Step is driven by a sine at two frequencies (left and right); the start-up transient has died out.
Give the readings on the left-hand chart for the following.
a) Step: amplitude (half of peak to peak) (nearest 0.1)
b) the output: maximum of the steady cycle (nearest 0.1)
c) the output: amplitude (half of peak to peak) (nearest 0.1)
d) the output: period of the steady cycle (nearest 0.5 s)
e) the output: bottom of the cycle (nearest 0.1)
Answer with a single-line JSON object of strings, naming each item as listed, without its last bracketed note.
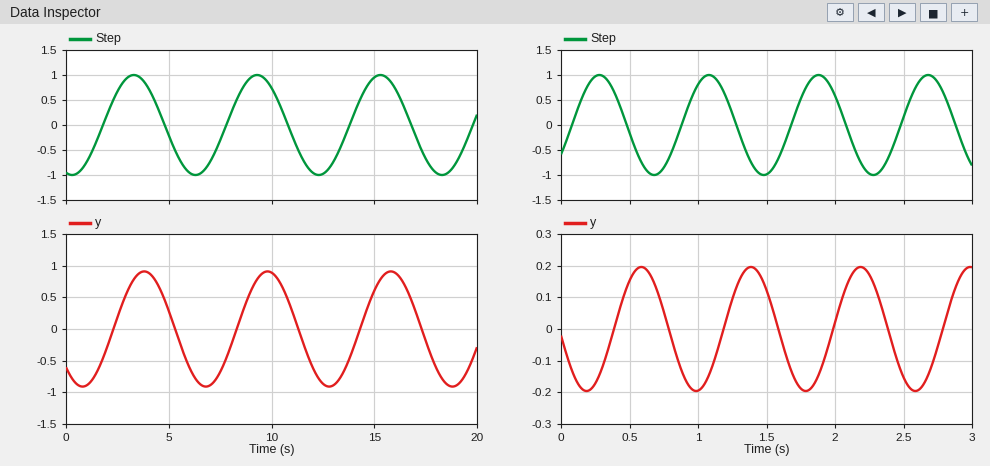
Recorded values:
{"Step: amplitude (half of peak to peak)": "1.0", "the output: maximum of the steady cycle": "0.9", "the output: amplitude (half of peak to peak)": "0.9", "the output: period of the steady cycle": "6.0 s", "the output: bottom of the cycle": "-0.9"}
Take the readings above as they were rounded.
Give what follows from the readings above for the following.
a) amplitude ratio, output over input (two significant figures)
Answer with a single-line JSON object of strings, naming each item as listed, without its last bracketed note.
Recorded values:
{"amplitude ratio, output over input": "0.90"}
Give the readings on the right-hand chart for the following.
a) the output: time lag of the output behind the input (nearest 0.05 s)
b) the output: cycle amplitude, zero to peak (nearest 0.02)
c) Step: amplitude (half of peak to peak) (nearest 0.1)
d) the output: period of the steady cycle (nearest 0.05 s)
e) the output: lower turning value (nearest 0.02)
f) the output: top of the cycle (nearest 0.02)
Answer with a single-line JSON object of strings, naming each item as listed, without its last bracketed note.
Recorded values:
{"the output: time lag of the output behind the input": "0.30 s", "the output: cycle amplitude, zero to peak": "0.20", "Step: amplitude (half of peak to peak)": "1.0", "the output: period of the steady cycle": "0.80 s", "the output: lower turning value": "-0.20", "the output: top of the cycle": "0.20"}
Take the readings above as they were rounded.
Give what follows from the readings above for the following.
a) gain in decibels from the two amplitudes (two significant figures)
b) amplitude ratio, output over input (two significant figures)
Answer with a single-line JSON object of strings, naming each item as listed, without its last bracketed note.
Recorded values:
{"gain in decibels from the two amplitudes": "-14 dB", "amplitude ratio, output over input": "0.20"}
